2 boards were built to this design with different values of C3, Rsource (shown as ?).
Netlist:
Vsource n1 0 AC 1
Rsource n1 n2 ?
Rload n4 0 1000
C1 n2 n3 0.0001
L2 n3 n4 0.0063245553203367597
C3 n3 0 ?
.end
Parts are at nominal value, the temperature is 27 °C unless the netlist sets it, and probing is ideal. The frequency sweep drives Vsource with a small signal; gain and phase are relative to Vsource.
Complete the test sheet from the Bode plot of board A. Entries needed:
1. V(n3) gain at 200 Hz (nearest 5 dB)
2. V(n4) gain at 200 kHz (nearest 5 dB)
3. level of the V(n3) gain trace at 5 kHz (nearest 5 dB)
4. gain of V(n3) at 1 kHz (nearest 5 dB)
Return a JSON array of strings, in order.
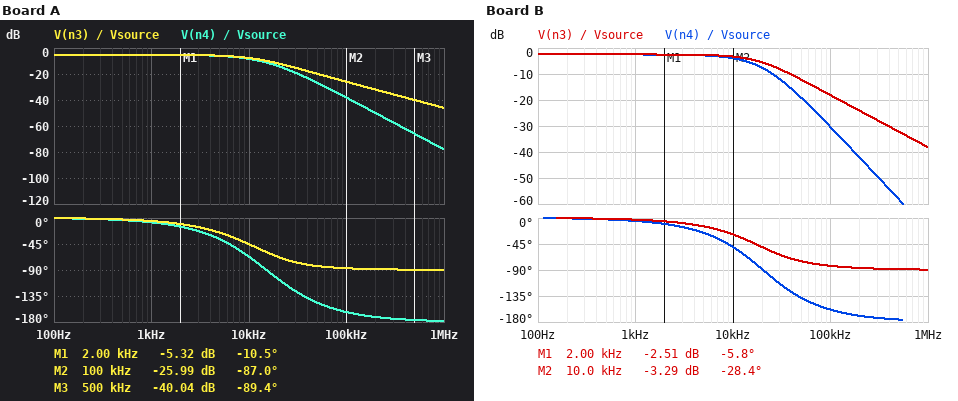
["-5 dB", "-50 dB", "-5 dB", "-5 dB"]
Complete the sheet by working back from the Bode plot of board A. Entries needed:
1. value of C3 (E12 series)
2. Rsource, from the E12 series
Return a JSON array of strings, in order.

["39 nF", "820 Ω"]
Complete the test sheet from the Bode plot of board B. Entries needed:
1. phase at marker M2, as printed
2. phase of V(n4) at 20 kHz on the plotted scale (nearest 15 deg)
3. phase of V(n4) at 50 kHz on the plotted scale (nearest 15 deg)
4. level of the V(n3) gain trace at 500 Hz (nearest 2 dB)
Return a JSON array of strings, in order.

["-28.4 deg", "-90 deg", "-135 deg", "-2 dB"]
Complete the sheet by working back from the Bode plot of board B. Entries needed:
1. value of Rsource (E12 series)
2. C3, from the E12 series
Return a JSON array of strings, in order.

["330 Ω", "39 nF"]
